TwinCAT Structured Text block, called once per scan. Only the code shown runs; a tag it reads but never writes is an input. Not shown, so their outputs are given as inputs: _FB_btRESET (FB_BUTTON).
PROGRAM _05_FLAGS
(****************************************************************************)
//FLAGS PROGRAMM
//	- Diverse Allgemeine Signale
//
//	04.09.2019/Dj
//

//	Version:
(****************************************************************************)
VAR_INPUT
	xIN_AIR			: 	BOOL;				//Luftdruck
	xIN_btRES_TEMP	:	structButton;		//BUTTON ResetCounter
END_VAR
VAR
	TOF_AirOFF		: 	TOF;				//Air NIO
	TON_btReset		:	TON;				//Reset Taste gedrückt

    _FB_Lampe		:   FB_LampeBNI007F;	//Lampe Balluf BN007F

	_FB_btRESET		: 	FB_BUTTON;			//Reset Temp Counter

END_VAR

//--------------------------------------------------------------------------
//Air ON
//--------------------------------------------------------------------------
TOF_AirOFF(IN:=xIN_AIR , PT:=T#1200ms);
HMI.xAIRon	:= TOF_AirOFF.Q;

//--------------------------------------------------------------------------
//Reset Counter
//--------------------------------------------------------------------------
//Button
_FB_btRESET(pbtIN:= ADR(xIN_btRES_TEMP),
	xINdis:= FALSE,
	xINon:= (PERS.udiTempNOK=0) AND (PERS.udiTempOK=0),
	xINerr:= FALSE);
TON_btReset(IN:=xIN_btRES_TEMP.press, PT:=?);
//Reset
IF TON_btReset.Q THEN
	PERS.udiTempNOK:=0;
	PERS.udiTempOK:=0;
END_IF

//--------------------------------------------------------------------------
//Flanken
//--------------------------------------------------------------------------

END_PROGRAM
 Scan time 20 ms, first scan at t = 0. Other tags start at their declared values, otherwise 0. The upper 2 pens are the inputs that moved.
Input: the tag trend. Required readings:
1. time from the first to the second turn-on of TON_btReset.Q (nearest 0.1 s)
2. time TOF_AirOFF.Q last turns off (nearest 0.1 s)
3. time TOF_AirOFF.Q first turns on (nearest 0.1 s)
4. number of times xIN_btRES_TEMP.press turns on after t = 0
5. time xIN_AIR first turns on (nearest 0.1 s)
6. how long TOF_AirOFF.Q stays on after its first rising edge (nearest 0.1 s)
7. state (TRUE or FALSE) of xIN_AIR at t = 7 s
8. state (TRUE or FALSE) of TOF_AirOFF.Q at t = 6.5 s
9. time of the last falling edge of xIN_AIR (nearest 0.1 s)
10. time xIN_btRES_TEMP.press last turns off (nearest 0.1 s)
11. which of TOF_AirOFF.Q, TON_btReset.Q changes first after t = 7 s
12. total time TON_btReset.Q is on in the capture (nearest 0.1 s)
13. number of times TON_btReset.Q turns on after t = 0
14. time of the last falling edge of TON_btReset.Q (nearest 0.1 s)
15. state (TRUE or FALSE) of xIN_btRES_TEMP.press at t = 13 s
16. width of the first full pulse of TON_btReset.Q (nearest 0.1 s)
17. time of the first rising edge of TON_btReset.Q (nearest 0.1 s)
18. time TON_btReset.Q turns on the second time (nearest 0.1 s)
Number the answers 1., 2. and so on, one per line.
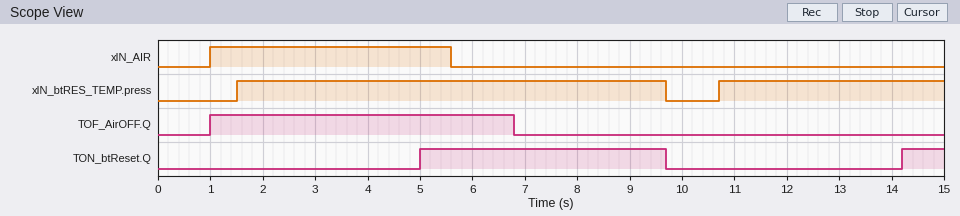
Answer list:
1. 9.2 s
2. 6.8 s
3. 1.0 s
4. 2
5. 1.0 s
6. 5.8 s
7. FALSE
8. TRUE
9. 5.6 s
10. 9.7 s
11. TON_btReset.Q
12. 5.5 s
13. 2
14. 9.7 s
15. TRUE
16. 4.7 s
17. 5.0 s
18. 14.2 s
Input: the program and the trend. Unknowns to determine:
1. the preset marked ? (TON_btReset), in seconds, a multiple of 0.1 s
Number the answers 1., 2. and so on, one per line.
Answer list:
1. 3.5 s
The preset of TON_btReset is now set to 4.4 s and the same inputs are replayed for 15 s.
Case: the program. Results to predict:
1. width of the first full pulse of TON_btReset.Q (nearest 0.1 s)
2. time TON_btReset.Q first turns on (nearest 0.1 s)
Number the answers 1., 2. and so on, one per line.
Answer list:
1. 3.8 s
2. 5.9 s
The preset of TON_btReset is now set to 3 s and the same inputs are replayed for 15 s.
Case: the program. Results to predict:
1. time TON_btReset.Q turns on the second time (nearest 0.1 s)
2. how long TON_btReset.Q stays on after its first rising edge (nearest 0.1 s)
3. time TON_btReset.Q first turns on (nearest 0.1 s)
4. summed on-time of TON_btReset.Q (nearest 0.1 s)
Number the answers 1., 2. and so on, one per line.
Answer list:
1. 13.7 s
2. 5.2 s
3. 4.5 s
4. 6.5 s
